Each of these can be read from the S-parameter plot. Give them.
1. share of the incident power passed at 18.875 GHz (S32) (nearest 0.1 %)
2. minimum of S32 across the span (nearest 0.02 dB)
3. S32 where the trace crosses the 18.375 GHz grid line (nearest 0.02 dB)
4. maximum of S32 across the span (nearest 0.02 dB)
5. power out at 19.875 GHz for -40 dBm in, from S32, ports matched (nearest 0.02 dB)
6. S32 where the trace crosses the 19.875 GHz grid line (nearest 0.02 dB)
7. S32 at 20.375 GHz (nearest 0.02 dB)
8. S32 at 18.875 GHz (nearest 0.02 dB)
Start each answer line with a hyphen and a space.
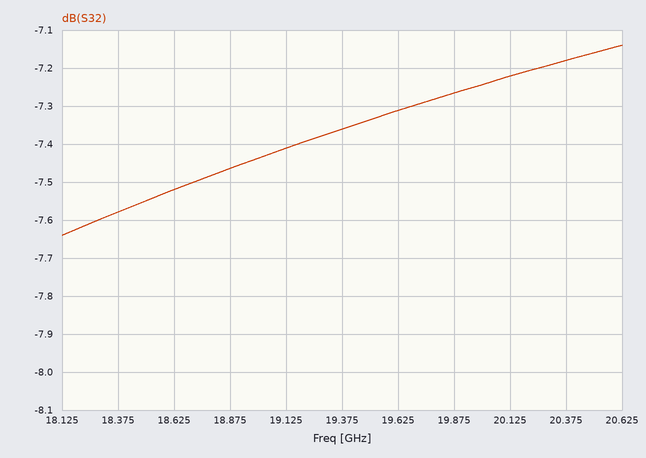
- 17.9 %
- -7.64 dB
- -7.58 dB
- -7.14 dB
- -47.26 dBm
- -7.26 dB
- -7.18 dB
- -7.46 dB
